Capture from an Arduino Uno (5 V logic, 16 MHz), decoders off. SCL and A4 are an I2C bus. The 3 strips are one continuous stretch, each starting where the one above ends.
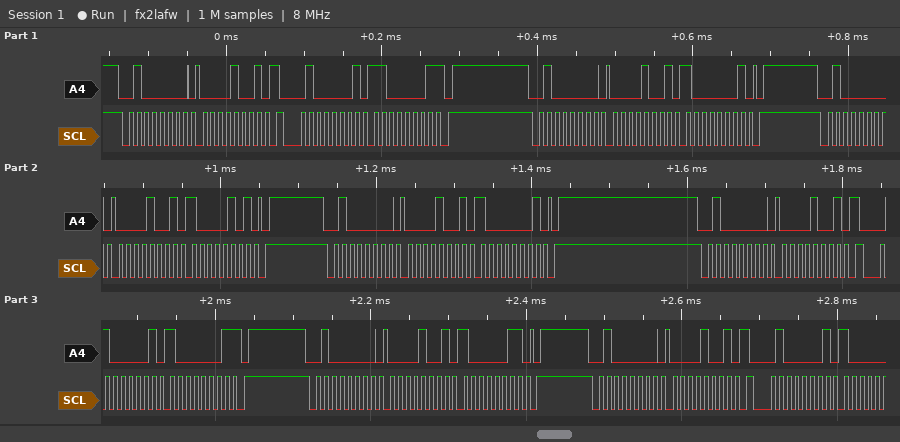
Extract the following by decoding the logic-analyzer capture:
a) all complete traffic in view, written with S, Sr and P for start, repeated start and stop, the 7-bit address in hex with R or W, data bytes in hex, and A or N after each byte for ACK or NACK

S 20W A 09 A Sr 20R A C1 N P S 20W A 09 A 81 A P S 20W A 09 A 85 A P S 20W A 09 A 81 A P S 20W A 09 A Sr 20R A 81 N P S 20W A 09 A 83 A P S 20W A 09 A Sr 20R A
